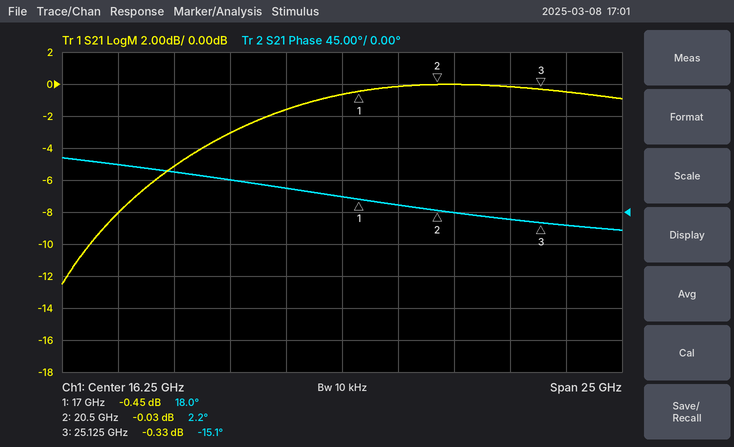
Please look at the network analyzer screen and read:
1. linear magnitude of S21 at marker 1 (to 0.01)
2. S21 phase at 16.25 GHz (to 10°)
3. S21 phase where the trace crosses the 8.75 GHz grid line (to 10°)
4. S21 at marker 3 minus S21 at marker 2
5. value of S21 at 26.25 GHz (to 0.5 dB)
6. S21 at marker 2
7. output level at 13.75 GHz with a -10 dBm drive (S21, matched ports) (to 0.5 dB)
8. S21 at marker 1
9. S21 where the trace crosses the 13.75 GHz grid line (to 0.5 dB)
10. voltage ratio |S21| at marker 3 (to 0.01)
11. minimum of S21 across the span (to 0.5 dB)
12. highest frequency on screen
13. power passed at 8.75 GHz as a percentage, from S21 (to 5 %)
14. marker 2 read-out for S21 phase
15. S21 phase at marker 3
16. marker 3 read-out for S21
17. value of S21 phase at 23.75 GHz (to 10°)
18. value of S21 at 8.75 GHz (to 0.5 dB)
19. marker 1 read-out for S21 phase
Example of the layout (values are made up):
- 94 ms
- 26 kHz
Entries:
- 0.95
- 20°
- 60°
- -0.30 dB
- -0.5 dB
- -0.03 dB
- -11.5 dBm
- -0.45 dB
- -1.5 dB
- 0.96
- -12.5 dB
- 28.75 GHz
- 30 %
- 2.2°
- -15.1°
- -0.33 dB
- -10°
- -5.0 dB
- 18.0°
